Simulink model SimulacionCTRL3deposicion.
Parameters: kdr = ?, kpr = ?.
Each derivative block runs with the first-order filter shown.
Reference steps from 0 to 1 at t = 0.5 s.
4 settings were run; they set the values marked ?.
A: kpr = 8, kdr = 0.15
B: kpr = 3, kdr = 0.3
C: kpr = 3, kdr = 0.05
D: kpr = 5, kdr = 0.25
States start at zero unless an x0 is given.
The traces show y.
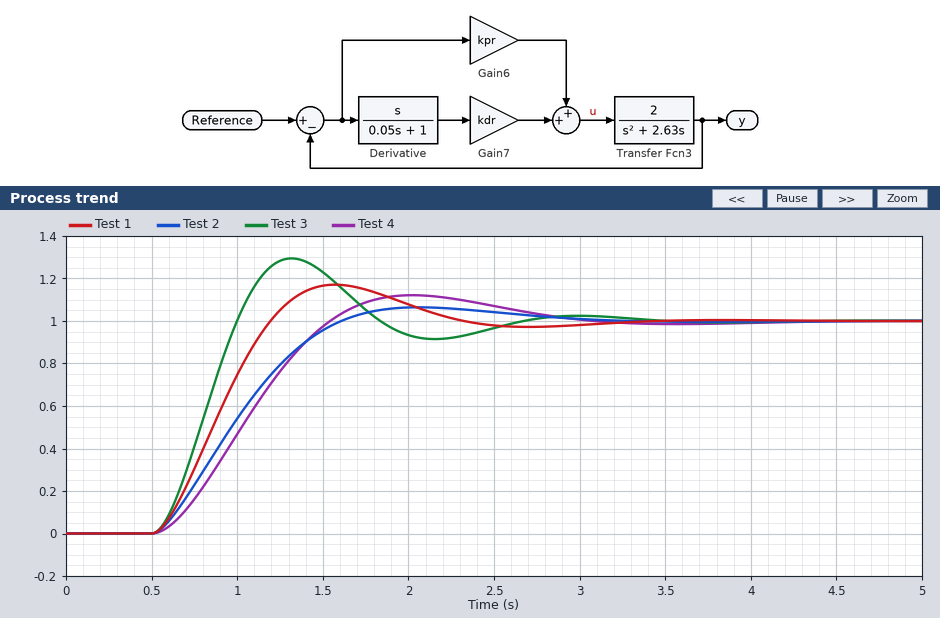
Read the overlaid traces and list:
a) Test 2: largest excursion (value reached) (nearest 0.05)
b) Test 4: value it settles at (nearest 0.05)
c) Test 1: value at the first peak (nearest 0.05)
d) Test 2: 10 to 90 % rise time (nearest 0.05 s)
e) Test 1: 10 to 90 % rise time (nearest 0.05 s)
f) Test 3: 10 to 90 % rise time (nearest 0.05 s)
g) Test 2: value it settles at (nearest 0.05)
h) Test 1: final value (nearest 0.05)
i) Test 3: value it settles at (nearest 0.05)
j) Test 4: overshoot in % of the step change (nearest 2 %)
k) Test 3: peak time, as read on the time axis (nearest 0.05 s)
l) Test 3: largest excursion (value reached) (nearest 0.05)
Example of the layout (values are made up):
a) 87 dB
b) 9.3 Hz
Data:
a) 1.05
b) 1.00
c) 1.15
d) 0.75 s
e) 0.50 s
f) 0.35 s
g) 1.00
h) 1.00
i) 1.00
j) 12 %
k) 1.30 s
l) 1.30
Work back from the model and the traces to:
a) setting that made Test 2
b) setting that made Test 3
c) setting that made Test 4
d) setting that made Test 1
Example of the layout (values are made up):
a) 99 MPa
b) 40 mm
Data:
a) B
b) A
c) C
d) D
